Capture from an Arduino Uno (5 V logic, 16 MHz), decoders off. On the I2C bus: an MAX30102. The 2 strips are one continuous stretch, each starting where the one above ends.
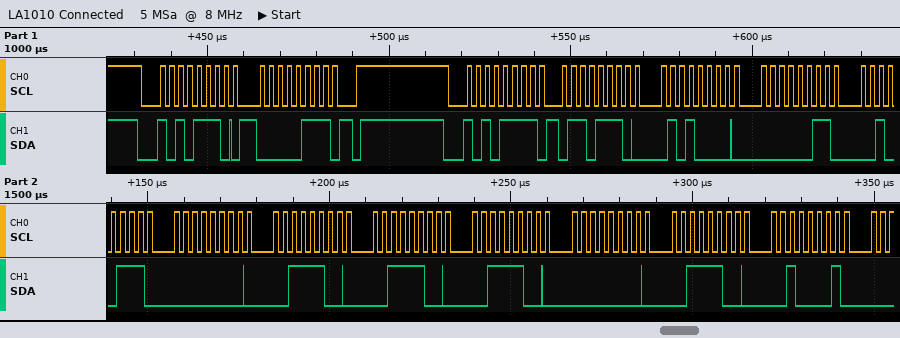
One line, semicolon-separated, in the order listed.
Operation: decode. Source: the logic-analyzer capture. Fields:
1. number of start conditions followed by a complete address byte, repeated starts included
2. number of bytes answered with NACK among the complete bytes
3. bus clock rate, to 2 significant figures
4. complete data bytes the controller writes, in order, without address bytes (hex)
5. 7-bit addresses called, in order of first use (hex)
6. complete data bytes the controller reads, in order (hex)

2; 0; 400 kHz; 07; 0x57; 6E 50 03 27 00 3C 3C 3C 00 3C 21
